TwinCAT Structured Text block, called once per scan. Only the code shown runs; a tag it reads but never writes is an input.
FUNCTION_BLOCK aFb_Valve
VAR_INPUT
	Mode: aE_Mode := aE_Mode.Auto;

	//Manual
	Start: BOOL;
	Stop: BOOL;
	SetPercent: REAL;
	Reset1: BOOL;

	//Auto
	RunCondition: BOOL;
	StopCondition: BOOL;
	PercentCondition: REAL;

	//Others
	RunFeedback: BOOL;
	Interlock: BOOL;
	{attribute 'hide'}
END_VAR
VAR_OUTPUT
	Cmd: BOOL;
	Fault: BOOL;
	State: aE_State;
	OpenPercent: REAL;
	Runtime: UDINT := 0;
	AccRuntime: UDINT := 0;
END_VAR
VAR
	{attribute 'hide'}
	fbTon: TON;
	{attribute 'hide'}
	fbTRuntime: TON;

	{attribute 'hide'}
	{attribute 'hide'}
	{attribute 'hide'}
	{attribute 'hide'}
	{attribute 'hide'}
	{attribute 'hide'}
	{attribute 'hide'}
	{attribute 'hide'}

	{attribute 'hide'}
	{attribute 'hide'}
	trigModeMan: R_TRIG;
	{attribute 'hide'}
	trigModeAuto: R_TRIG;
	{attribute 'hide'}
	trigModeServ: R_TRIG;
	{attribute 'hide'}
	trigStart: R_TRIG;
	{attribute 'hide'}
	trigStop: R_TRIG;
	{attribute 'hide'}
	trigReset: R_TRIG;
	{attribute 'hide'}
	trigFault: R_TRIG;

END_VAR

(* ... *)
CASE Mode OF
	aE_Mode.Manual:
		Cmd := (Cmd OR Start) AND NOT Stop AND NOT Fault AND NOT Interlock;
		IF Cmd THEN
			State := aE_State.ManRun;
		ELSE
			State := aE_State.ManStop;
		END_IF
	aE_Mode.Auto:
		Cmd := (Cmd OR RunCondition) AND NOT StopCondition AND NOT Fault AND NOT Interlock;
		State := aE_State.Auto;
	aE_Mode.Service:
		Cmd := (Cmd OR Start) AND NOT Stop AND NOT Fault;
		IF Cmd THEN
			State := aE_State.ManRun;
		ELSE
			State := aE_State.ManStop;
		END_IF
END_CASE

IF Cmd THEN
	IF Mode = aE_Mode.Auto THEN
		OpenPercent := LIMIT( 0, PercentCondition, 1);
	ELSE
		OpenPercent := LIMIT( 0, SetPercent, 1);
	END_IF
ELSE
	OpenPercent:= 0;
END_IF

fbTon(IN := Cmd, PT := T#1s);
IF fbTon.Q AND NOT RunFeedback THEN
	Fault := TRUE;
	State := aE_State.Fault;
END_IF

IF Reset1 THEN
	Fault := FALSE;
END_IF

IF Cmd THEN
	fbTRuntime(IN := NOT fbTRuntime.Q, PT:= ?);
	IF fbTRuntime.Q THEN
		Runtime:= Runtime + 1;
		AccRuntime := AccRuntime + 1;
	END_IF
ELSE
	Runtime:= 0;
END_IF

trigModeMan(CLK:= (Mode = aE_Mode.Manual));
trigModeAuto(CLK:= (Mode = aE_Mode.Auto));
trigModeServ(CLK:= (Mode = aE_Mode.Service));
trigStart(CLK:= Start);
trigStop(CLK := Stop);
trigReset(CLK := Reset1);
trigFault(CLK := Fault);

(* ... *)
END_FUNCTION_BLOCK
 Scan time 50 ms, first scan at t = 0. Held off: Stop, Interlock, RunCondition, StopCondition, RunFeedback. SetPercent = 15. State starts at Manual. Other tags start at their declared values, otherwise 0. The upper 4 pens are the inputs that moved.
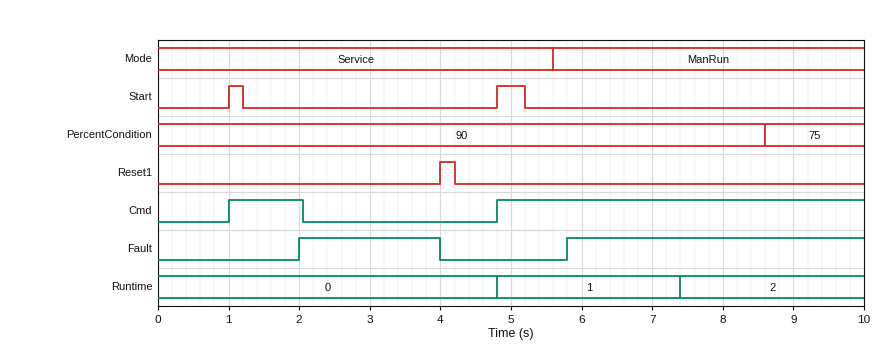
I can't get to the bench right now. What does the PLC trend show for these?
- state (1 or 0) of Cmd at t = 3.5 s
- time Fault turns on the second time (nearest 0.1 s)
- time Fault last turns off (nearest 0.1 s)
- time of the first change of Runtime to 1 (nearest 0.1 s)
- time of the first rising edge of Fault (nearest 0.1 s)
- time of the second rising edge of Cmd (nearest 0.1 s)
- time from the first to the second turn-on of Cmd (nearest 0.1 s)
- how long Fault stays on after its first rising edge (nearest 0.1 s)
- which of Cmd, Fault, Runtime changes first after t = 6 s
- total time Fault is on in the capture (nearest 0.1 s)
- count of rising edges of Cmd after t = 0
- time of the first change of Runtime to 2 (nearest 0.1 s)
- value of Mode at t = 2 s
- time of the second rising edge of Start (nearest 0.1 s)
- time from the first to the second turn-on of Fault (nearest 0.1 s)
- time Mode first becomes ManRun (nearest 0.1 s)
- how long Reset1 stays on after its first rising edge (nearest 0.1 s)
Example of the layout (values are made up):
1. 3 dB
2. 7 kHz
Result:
1. 0
2. 5.8 s
3. 4.0 s
4. 4.8 s
5. 2.0 s
6. 4.8 s
7. 3.8 s
8. 2.0 s
9. Runtime
10. 6.2 s
11. 2
12. 7.4 s
13. Service
14. 4.8 s
15. 3.8 s
16. 5.6 s
17. 0.2 s
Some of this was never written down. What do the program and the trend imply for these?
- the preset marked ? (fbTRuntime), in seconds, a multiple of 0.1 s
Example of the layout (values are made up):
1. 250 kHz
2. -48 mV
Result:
1. 2.5 s
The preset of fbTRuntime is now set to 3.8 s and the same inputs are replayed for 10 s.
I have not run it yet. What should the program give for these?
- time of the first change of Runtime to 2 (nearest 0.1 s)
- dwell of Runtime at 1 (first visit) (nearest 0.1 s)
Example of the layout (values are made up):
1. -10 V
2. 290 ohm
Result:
1. 8.7 s
2. 3.9 s
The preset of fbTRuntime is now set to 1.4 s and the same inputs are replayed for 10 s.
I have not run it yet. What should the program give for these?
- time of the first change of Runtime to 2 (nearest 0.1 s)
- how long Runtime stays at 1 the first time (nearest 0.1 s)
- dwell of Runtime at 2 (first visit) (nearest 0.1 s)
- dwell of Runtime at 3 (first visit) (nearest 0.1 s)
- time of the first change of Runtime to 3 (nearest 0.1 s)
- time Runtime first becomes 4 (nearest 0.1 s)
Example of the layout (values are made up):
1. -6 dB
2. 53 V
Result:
1. 6.3 s
2. 1.5 s
3. 1.5 s
4. 1.5 s
5. 7.8 s
6. 9.3 s
